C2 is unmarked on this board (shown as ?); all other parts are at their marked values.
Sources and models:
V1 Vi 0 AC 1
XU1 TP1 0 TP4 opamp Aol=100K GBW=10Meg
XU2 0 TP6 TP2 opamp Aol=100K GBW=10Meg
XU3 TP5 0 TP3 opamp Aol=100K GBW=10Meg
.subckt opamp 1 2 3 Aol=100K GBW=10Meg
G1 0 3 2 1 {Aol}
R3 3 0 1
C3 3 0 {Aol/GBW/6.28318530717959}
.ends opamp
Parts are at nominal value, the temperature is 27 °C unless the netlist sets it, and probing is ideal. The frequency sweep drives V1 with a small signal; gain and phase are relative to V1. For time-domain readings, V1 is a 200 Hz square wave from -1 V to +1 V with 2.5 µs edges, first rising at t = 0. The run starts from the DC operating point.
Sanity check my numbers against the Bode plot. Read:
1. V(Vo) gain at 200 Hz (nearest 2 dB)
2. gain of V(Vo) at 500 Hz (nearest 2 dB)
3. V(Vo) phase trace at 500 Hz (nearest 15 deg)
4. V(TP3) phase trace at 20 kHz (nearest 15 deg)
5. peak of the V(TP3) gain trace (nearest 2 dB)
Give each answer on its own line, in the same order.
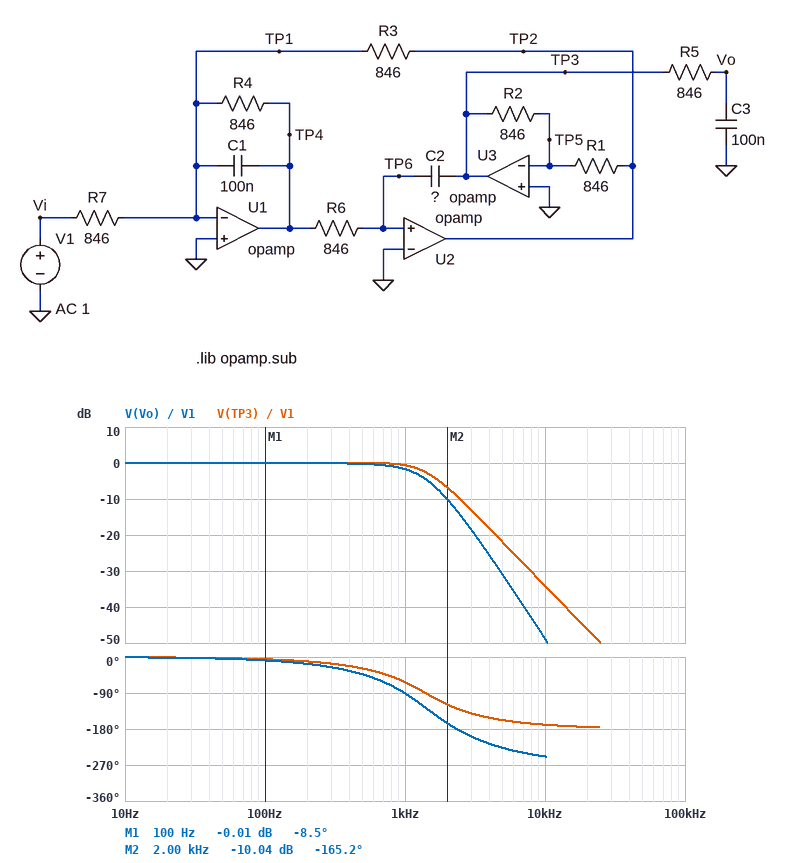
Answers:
0 dB
0 dB
-45 deg
-180 deg
0 dB
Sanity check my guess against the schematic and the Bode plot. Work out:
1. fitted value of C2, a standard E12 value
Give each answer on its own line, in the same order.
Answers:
180 nF
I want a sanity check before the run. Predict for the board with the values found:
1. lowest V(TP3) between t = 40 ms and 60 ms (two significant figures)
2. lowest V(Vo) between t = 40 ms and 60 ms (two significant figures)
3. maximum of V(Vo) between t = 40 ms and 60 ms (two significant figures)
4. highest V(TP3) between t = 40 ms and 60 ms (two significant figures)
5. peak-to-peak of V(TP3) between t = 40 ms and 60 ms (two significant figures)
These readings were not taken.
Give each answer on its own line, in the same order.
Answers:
-1.1 V
-1.1 V
1.1 V
1.1 V
2.2 V
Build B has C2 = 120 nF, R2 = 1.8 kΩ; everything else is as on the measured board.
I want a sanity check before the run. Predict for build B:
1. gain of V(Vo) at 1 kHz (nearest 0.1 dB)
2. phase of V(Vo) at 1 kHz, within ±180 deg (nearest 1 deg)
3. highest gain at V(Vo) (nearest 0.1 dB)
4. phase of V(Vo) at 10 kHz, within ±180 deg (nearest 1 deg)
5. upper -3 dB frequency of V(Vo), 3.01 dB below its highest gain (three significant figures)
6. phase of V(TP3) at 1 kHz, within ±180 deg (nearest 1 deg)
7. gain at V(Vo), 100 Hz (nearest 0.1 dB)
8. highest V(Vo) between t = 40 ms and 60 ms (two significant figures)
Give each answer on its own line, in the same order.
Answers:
2.6 dB
-106 deg
6.6 dB
111 deg
887 Hz
-78 deg
6.5 dB
2.2 V
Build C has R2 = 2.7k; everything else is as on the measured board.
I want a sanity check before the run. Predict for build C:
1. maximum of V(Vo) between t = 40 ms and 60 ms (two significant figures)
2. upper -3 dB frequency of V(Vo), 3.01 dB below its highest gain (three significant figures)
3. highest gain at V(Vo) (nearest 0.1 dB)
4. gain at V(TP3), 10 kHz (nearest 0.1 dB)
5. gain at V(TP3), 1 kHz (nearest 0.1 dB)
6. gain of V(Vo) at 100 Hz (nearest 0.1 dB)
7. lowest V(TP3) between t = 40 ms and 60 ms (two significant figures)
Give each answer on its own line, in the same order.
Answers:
3.2 V
378 Hz
10.1 dB
-34.2 dB
0.2 dB
9.8 dB
-3.2 V
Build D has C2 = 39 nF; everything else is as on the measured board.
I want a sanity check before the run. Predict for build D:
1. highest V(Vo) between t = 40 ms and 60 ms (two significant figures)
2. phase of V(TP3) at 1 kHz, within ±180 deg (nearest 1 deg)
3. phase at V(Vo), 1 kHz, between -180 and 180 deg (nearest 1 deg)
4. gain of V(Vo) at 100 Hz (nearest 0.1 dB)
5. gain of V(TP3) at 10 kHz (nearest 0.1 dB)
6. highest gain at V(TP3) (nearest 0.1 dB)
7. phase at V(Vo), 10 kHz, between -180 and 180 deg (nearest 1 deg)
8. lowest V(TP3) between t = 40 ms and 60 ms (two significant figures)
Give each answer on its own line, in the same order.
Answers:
1.2 V
-13 deg
-41 deg
0 dB
-20.2 dB
4.5 dB
112 deg
-1.7 V
